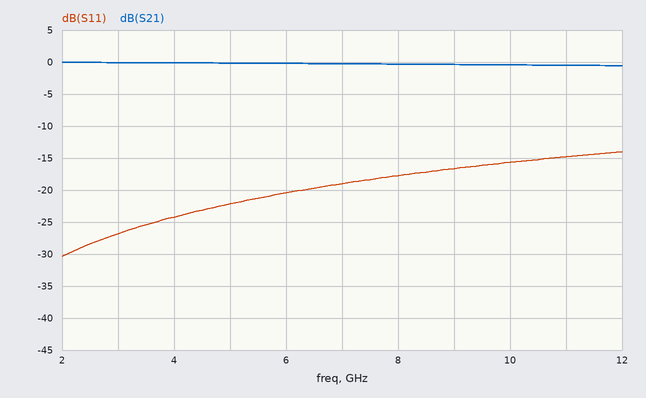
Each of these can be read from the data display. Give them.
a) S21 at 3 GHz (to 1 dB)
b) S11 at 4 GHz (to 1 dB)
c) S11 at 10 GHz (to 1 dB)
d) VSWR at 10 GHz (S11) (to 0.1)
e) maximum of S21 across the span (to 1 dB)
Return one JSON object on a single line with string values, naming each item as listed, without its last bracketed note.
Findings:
{"S21 at 3 GHz": "0 dB", "S11 at 4 GHz": "-24 dB", "S11 at 10 GHz": "-16 dB", "VSWR at 10 GHz (S11)": "1.4", "maximum of S21 across the span": "0 dB"}
